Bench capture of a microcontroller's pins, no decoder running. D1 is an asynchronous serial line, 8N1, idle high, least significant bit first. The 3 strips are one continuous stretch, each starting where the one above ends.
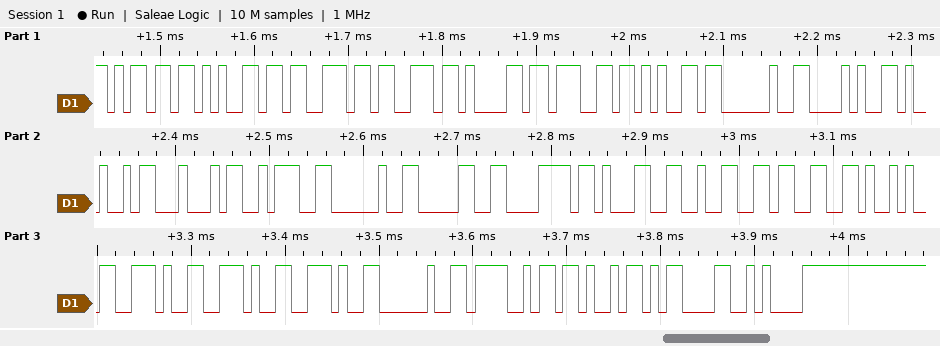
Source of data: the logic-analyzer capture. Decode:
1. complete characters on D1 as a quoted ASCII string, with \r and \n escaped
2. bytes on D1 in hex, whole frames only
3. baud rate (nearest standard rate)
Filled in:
"message (ID: 0x123)... OK\r\n"
6D 65 73 73 61 67 65 20 28 49 44 3A 20 30 78 31 32 33 29 2E 2E 2E 20 4F 4B 0D 0A
115200 baud
